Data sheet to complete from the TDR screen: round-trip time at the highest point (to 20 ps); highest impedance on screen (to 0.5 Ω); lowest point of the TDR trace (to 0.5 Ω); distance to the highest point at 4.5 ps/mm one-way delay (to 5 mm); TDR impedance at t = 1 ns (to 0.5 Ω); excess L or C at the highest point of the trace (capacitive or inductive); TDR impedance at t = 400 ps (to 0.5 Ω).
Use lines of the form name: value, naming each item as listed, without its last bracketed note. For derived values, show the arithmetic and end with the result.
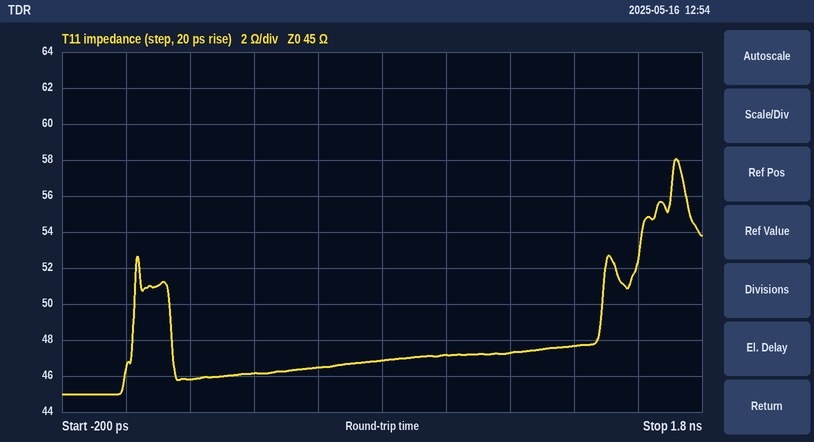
round-trip time at the highest point: 1.72 ns
highest impedance on screen: 58.0 Ω
lowest point of the TDR trace: 45.0 Ω
distance to the highest point at 4.5 ps/mm one-way delay: 1.72 ns / 2 / 4.5 ps/mm ≈ 191 mm, so 190 mm to the nearest 5 mm
TDR impedance at t = 1 ns: 47.0 Ω
excess L or C at the highest point of the trace: inductive
TDR impedance at t = 400 ps: 46.0 Ω
